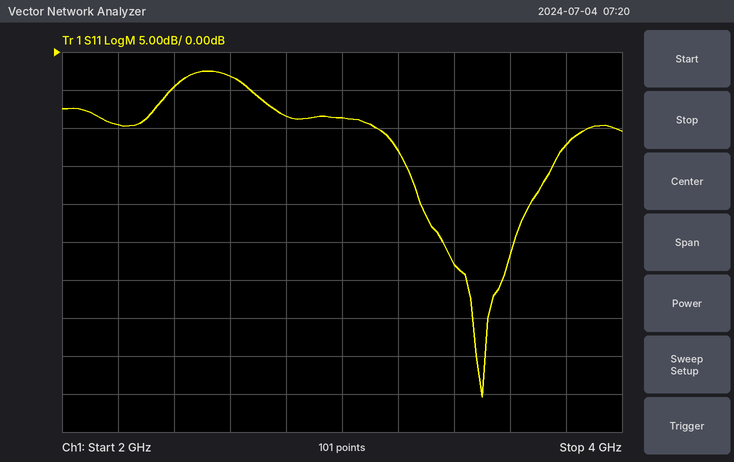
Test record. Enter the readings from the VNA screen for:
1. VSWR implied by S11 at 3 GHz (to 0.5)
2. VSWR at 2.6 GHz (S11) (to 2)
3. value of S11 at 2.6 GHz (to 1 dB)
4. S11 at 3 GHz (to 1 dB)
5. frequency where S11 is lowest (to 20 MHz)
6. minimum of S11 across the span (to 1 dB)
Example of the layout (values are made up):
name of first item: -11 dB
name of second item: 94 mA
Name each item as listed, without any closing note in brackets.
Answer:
VSWR implied by S11 at 3 GHz: 2.0
VSWR at 2.6 GHz (S11): 6
value of S11 at 2.6 GHz: -3 dB
S11 at 3 GHz: -9 dB
frequency where S11 is lowest: 3.50 GHz
minimum of S11 across the span: -45 dB
